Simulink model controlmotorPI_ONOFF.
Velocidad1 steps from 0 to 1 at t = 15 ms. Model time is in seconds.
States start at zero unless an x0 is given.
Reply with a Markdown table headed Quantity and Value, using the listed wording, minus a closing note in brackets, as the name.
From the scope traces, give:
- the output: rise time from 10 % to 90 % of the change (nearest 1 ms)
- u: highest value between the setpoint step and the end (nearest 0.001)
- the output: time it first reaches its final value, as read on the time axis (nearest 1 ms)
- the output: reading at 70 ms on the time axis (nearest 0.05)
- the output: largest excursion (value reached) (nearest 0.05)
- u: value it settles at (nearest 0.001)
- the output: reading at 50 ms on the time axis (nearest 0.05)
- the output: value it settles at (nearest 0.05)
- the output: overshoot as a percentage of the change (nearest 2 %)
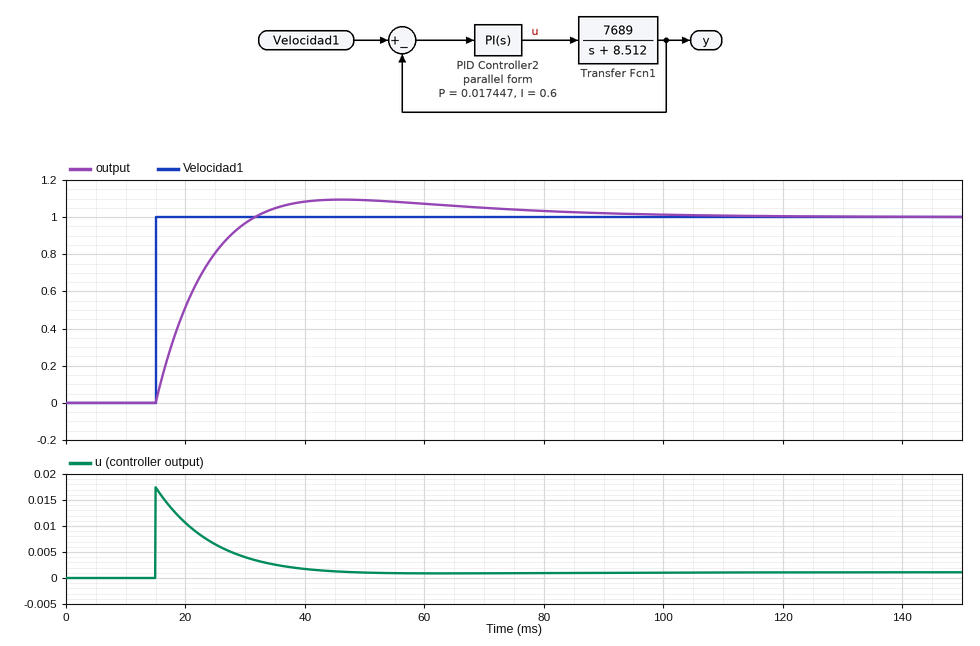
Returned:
| Quantity | Value |
|---|---|
| the output: rise time from 10 % to 90 % of the change | 12 ms |
| u: highest value between the setpoint step and the end | 0.017 |
| the output: time it first reaches its final value, as read on the time axis | 32 ms |
| the output: reading at 70 ms on the time axis | 1.05 |
| the output: largest excursion (value reached) | 1.10 |
| u: value it settles at | 0.001 |
| the output: reading at 50 ms on the time axis | 1.10 |
| the output: value it settles at | 1.00 |
| the output: overshoot as a percentage of the change | 10 % |
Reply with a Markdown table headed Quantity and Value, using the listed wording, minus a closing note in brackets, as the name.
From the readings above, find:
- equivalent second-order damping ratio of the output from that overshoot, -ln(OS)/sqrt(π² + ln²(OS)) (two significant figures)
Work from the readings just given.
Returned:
| Quantity | Value |
|---|---|
| equivalent second-order damping ratio of the output from that overshoot, -ln(OS)/sqrt(π² + ln²(OS)) | 0.59 |
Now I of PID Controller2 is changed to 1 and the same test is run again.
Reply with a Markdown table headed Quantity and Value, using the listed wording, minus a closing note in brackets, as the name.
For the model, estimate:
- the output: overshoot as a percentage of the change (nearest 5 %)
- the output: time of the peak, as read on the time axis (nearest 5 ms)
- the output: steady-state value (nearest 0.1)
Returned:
| Quantity | Value |
|---|---|
| the output: overshoot as a percentage of the change | 15 % |
| the output: time of the peak, as read on the time axis | 40 ms |
| the output: steady-state value | 1.0 |
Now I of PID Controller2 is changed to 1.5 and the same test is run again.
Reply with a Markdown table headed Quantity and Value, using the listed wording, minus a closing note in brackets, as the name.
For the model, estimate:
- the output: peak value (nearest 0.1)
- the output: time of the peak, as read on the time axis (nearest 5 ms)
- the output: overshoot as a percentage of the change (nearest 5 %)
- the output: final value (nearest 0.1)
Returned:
| Quantity | Value |
|---|---|
| the output: peak value | 1.2 |
| the output: time of the peak, as read on the time axis | 35 ms |
| the output: overshoot as a percentage of the change | 20 % |
| the output: final value | 1.0 |
